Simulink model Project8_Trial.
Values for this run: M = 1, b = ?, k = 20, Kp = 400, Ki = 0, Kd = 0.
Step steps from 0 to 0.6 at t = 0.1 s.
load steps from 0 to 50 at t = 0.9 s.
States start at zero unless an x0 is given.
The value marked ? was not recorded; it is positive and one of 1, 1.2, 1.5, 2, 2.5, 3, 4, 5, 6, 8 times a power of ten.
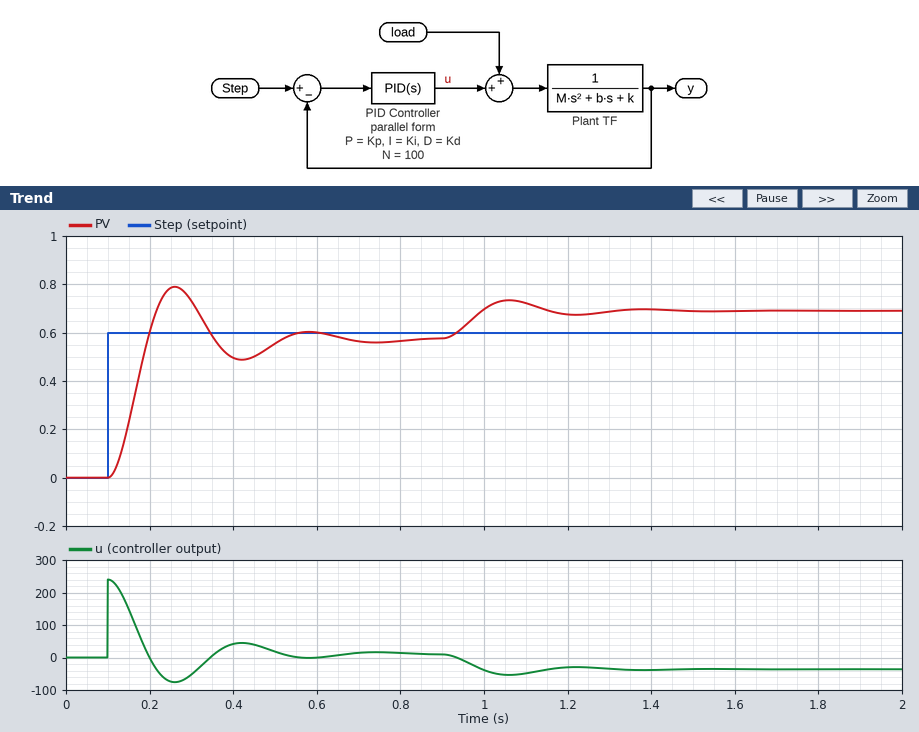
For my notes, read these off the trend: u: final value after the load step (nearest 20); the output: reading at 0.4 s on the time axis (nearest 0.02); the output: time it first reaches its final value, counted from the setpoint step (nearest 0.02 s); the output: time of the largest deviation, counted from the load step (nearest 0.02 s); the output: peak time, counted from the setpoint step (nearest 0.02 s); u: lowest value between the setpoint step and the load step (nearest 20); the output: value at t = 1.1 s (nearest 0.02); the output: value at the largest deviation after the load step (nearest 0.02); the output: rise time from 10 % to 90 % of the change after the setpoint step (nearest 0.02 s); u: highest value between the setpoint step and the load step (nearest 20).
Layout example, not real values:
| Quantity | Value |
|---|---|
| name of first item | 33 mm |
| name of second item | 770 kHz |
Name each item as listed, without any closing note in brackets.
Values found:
| Quantity | Value |
|---|---|
| u: final value after the load step | -40 |
| the output: reading at 0.4 s on the time axis | 0.50 |
| the output: time it first reaches its final value, counted from the setpoint step | 0.10 s |
| the output: time of the largest deviation, counted from the load step | 0.16 s |
| the output: peak time, counted from the setpoint step | 0.16 s |
| u: lowest value between the setpoint step and the load step | -80 |
| the output: value at t = 1.1 s | 0.72 |
| the output: value at the largest deviation after the load step | 0.74 |
| the output: rise time from 10 % to 90 % of the change after the setpoint step | 0.06 s |
| u: highest value between the setpoint step and the load step | 240 |
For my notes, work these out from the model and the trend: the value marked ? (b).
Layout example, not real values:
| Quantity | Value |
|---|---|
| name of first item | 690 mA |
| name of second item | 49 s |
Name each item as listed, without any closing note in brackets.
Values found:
| Quantity | Value |
|---|---|
| the value marked ? | 12 |
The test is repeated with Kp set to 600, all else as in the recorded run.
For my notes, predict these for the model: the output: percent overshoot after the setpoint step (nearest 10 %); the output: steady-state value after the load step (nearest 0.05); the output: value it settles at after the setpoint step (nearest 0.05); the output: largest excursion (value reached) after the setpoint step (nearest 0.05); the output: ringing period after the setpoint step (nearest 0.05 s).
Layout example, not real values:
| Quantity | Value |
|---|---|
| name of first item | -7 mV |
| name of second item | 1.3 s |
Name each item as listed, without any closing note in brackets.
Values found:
| Quantity | Value |
|---|---|
| the output: percent overshoot after the setpoint step | 50 % |
| the output: steady-state value after the load step | 0.65 |
| the output: value it settles at after the setpoint step | 0.60 |
| the output: largest excursion (value reached) after the setpoint step | 0.85 |
| the output: ringing period after the setpoint step | 0.25 s |
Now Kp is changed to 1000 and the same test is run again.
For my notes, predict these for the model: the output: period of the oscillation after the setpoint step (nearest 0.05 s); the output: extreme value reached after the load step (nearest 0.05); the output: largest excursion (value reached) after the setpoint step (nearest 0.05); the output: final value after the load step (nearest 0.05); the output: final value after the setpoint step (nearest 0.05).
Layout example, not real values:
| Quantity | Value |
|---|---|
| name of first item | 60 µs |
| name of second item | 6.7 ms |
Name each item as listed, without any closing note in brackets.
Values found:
| Quantity | Value |
|---|---|
| the output: period of the oscillation after the setpoint step | 0.20 s |
| the output: extreme value reached after the load step | 0.65 |
| the output: largest excursion (value reached) after the setpoint step | 0.90 |
| the output: final value after the load step | 0.65 |
| the output: final value after the setpoint step | 0.60 |
